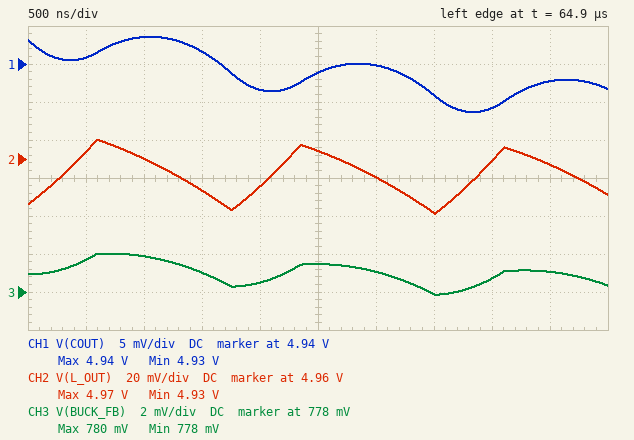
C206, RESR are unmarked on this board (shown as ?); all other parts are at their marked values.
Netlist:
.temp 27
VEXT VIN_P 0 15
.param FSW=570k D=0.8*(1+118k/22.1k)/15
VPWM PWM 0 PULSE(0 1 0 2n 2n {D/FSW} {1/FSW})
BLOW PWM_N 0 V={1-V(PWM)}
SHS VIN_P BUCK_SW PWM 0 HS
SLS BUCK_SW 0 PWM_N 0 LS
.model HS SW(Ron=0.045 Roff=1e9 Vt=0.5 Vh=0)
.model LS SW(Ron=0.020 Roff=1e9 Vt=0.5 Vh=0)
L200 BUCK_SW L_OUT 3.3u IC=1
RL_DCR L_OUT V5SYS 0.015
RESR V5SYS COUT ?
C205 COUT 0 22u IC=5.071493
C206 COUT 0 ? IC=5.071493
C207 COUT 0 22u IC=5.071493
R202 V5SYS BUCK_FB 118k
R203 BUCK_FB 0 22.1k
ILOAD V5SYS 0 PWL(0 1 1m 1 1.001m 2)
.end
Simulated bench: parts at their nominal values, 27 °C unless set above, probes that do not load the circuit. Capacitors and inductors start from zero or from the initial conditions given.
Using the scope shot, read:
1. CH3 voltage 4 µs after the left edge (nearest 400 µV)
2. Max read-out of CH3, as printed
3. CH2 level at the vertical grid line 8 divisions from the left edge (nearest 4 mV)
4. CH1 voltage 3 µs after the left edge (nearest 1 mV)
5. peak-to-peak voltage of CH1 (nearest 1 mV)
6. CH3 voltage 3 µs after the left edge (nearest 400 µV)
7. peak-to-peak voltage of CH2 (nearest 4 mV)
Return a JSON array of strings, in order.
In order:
["778.8 mV", "780 mV", "4.960 V", "4.940 V", "10 mV", "779.2 mV", "40 mV"]
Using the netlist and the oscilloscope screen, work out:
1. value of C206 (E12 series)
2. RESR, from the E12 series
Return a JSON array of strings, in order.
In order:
["33 µF", "4.7 mΩ"]
